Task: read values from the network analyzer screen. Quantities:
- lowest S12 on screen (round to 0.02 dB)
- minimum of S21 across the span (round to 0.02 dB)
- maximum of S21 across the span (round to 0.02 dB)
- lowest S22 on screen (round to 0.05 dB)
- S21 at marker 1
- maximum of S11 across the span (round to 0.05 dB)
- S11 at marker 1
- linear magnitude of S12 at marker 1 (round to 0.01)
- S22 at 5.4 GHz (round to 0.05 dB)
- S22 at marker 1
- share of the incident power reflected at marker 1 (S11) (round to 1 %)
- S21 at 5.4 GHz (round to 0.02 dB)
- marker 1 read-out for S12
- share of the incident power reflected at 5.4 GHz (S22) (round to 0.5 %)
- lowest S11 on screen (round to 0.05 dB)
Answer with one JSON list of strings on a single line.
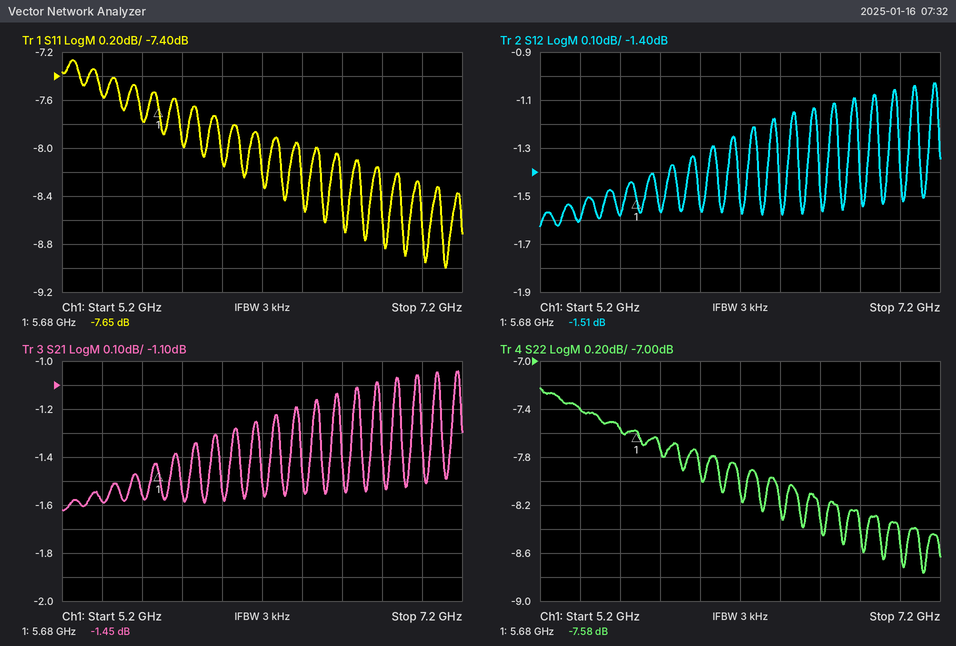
["-1.62 dB", "-1.62 dB", "-1.04 dB", "-8.75 dB", "-1.45 dB", "-7.25 dB", "-7.65 dB", "0.84", "-7.40 dB", "-7.58 dB", "17 %", "-1.58 dB", "-1.51 dB", "18.0 %", "-9.00 dB"]
